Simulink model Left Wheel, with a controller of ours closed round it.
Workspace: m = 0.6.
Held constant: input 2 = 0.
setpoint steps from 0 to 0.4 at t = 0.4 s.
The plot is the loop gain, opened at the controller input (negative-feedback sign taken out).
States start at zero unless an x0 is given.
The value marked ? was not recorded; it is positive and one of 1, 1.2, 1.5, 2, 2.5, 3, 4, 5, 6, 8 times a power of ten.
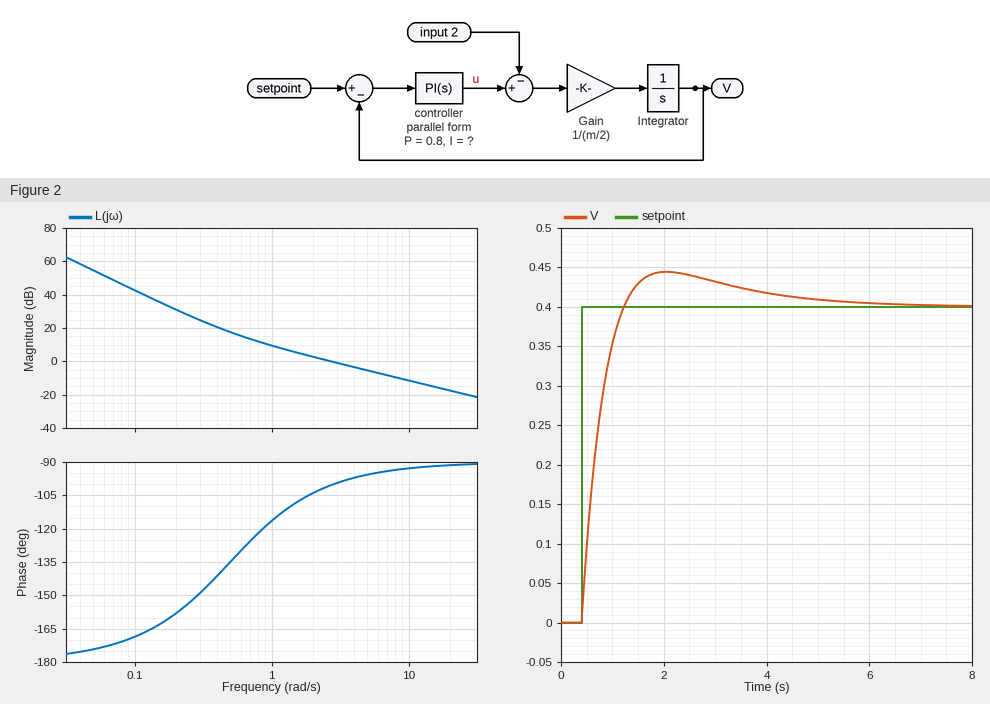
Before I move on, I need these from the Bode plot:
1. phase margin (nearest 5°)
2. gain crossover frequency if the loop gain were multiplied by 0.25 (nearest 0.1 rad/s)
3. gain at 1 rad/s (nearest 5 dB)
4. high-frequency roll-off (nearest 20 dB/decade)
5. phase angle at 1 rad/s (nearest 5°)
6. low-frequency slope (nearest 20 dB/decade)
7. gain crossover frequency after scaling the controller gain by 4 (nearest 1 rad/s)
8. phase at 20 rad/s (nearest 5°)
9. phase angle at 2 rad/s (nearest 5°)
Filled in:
80°
0.8 rad/s
10 dB
-20 dB/decade
-115°
-40 dB/decade
11 rad/s
-90°
-105°
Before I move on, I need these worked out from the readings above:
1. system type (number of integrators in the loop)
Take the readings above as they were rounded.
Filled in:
2
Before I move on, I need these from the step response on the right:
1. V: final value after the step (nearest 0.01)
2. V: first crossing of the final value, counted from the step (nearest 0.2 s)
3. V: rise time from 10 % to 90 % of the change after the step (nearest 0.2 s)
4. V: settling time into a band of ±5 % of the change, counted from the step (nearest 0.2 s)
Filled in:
0.40
0.8 s
0.6 s
3.4 s
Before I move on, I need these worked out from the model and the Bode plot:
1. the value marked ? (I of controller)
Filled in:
0.4
